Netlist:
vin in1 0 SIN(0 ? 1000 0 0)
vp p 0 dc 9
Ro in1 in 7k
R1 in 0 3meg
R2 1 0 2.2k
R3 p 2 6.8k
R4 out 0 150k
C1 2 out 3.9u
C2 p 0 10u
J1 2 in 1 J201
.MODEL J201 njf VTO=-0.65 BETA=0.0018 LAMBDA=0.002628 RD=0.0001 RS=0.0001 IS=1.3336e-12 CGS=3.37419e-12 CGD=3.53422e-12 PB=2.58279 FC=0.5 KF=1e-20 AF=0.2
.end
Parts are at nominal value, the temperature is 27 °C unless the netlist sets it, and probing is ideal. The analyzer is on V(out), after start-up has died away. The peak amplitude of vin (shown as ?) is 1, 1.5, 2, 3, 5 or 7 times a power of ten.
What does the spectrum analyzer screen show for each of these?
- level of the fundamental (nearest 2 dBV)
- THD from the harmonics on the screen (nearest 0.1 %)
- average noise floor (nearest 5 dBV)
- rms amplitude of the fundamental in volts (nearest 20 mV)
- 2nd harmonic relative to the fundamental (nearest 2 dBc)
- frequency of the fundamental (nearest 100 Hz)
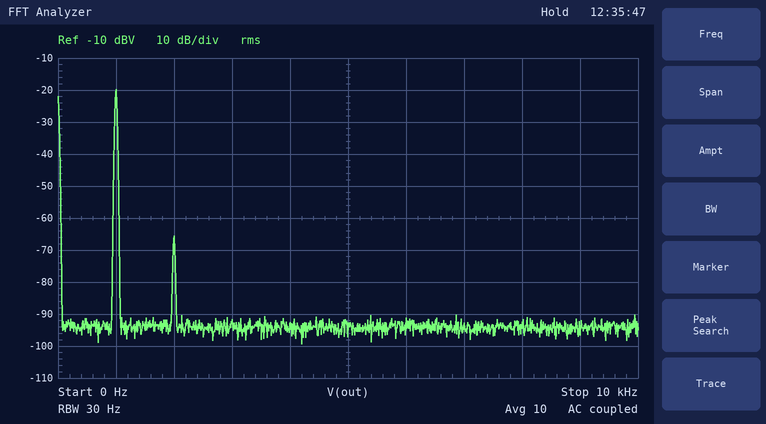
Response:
-20 dBV
0.5 %
-95 dBV
100 mV
-46 dBc
1.0 kHz
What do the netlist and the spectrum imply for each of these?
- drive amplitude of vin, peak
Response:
70 mV
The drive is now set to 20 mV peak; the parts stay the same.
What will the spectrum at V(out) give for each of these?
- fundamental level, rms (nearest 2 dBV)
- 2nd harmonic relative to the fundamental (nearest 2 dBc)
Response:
-30 dBV
-56 dBc
